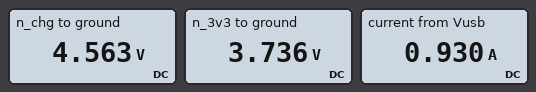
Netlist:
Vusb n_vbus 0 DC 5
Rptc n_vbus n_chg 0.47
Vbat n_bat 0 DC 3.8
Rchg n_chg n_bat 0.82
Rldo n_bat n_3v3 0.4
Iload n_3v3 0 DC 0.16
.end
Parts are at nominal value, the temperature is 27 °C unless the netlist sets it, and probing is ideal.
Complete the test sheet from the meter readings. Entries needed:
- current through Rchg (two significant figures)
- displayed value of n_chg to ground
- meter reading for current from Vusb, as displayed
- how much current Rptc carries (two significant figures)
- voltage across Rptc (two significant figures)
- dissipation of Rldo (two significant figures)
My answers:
930 mA
4.563 V
0.930 A
930 mA
440 mV
10 mW
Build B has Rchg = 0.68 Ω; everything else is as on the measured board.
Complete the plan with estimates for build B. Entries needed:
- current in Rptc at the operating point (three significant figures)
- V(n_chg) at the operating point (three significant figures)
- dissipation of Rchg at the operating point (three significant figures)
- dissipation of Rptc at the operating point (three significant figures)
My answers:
1.04 A
4.51 V
740 mW
512 mW
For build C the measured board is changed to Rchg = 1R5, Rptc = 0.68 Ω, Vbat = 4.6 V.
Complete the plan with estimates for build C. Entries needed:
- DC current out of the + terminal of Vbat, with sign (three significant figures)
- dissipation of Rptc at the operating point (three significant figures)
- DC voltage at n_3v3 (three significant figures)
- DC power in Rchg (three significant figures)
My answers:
-23.5 mA
22.9 mW
4.54 V
50.5 mW
